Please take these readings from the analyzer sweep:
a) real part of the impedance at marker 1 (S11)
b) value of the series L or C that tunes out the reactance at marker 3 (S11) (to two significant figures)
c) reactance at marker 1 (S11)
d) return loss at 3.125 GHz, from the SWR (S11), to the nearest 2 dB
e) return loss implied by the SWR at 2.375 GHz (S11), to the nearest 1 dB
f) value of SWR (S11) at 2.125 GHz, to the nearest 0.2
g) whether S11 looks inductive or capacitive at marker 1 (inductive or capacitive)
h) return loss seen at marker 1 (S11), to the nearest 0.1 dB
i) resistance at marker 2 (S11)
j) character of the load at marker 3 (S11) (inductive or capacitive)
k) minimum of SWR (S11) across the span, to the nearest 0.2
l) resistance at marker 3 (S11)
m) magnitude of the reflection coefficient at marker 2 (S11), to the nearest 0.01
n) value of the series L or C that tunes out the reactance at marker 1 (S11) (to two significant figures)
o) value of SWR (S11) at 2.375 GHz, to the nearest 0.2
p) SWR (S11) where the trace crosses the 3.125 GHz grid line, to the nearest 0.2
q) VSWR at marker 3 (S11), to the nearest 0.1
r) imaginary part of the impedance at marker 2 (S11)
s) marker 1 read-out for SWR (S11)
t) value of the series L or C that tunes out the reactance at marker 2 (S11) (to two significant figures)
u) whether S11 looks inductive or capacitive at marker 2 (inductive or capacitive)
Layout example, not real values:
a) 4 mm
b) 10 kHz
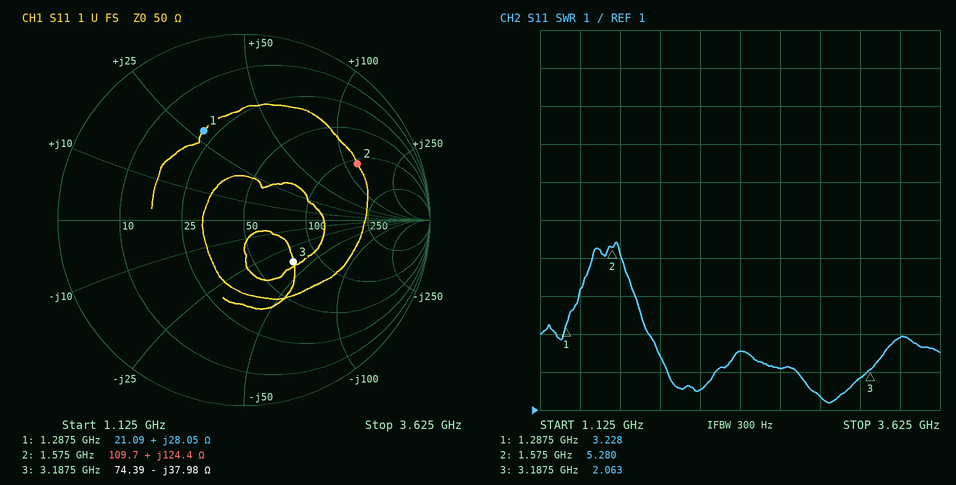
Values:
a) 21.09 Ω
b) 1.9 nH
c) +28.05 Ω
d) 10 dB
e) 7 dB
f) 1.6
g) inductive
h) 5.6 dB
i) 109.7 Ω
j) capacitive
k) 1.2
l) 74.39 Ω
m) 0.68
n) 4.4 pF
o) 2.6
p) 1.8
q) 2.1
r) +124.4 Ω
s) 3.228
t) 810 fF
u) inductive
